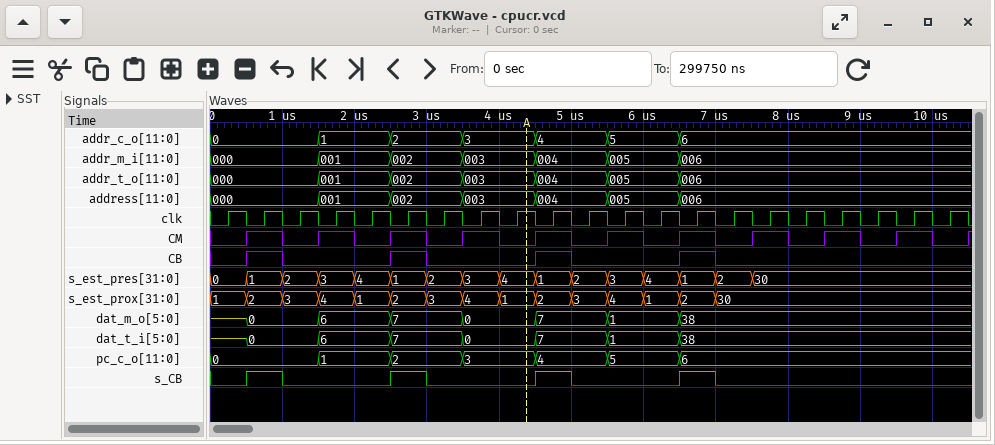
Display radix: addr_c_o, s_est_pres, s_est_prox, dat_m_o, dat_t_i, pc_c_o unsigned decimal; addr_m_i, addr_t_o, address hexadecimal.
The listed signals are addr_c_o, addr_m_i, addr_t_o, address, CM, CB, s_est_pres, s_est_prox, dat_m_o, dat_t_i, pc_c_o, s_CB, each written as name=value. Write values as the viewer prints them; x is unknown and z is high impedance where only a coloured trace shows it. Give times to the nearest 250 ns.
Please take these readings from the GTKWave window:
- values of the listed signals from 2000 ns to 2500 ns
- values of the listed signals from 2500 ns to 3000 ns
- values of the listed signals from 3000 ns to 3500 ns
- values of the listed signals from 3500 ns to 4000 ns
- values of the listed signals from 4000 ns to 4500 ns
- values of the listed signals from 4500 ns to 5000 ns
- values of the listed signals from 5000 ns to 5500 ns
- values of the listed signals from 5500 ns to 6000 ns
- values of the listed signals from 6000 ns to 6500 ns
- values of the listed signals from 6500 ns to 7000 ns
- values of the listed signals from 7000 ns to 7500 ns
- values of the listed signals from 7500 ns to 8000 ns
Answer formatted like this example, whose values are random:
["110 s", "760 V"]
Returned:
["addr_c_o=1, addr_m_i=001, addr_t_o=001, address=001, CM=0, CB=0, s_est_pres=4, s_est_prox=1, dat_m_o=6, dat_t_i=6, pc_c_o=1, s_CB=0", "addr_c_o=2, addr_m_i=002, addr_t_o=002, address=002, CM=1, CB=1, s_est_pres=1, s_est_prox=2, dat_m_o=7, dat_t_i=7, pc_c_o=2, s_CB=1", "addr_c_o=2, addr_m_i=002, addr_t_o=002, address=002, CM=0, CB=0, s_est_pres=2, s_est_prox=3, dat_m_o=7, dat_t_i=7, pc_c_o=2, s_CB=0", "addr_c_o=3, addr_m_i=003, addr_t_o=003, address=003, CM=1, CB=0, s_est_pres=3, s_est_prox=4, dat_m_o=0, dat_t_i=0, pc_c_o=3, s_CB=0", "addr_c_o=3, addr_m_i=003, addr_t_o=003, address=003, CM=0, CB=0, s_est_pres=4, s_est_prox=1, dat_m_o=0, dat_t_i=0, pc_c_o=3, s_CB=0", "addr_c_o=4, addr_m_i=004, addr_t_o=004, address=004, CM=1, CB=1, s_est_pres=1, s_est_prox=2, dat_m_o=7, dat_t_i=7, pc_c_o=4, s_CB=1", "addr_c_o=4, addr_m_i=004, addr_t_o=004, address=004, CM=0, CB=0, s_est_pres=2, s_est_prox=3, dat_m_o=7, dat_t_i=7, pc_c_o=4, s_CB=0", "addr_c_o=5, addr_m_i=005, addr_t_o=005, address=005, CM=1, CB=0, s_est_pres=3, s_est_prox=4, dat_m_o=1, dat_t_i=1, pc_c_o=5, s_CB=0", "addr_c_o=5, addr_m_i=005, addr_t_o=005, address=005, CM=0, CB=0, s_est_pres=4, s_est_prox=1, dat_m_o=1, dat_t_i=1, pc_c_o=5, s_CB=0", "addr_c_o=6, addr_m_i=006, addr_t_o=006, address=006, CM=1, CB=1, s_est_pres=1, s_est_prox=2, dat_m_o=38, dat_t_i=38, pc_c_o=6, s_CB=1", "addr_c_o=6, addr_m_i=006, addr_t_o=006, address=006, CM=0, CB=0, s_est_pres=2, s_est_prox=30, dat_m_o=38, dat_t_i=38, pc_c_o=6, s_CB=0", "addr_c_o=6, addr_m_i=006, addr_t_o=006, address=006, CM=1, CB=0, s_est_pres=30, s_est_prox=30, dat_m_o=38, dat_t_i=38, pc_c_o=6, s_CB=0"]
